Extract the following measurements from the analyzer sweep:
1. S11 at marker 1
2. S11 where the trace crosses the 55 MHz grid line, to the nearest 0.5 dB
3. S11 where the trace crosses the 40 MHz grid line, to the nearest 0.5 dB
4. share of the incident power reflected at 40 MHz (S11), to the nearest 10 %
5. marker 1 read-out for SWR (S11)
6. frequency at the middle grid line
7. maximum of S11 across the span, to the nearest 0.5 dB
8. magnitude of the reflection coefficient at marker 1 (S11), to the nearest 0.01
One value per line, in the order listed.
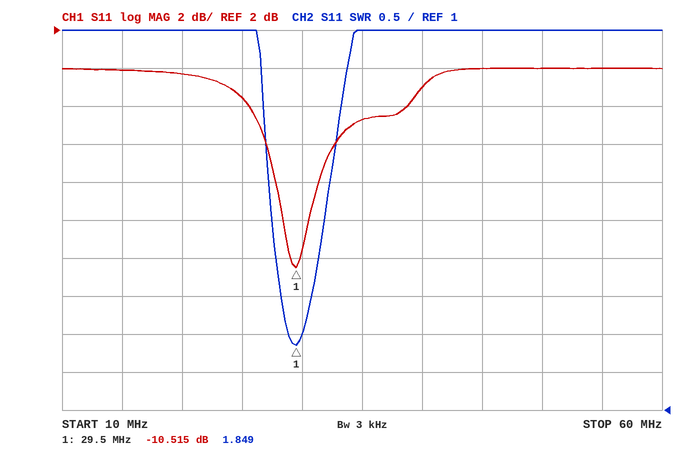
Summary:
-10.515 dB
0.0 dB
-1.0 dB
80 %
1.849
35 MHz
0.0 dB
0.30
